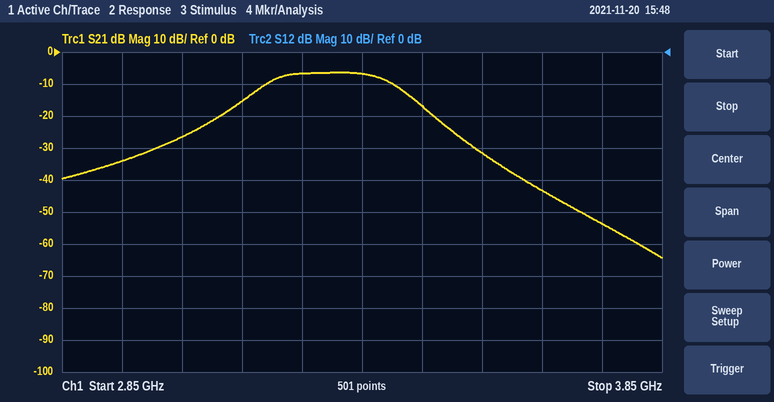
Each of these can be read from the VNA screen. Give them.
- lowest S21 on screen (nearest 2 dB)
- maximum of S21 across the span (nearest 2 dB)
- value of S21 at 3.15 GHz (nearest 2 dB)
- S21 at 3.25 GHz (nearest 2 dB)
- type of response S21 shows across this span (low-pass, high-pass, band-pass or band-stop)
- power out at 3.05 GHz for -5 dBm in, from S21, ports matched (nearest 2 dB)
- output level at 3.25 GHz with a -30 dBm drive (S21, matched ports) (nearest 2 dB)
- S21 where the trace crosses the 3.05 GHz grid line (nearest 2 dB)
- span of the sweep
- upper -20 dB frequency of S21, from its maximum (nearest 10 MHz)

-64 dB
-6 dB
-16 dB
-6 dB
band-pass
-32 dBm
-36 dBm
-26 dB
1 GHz
3.51 GHz
